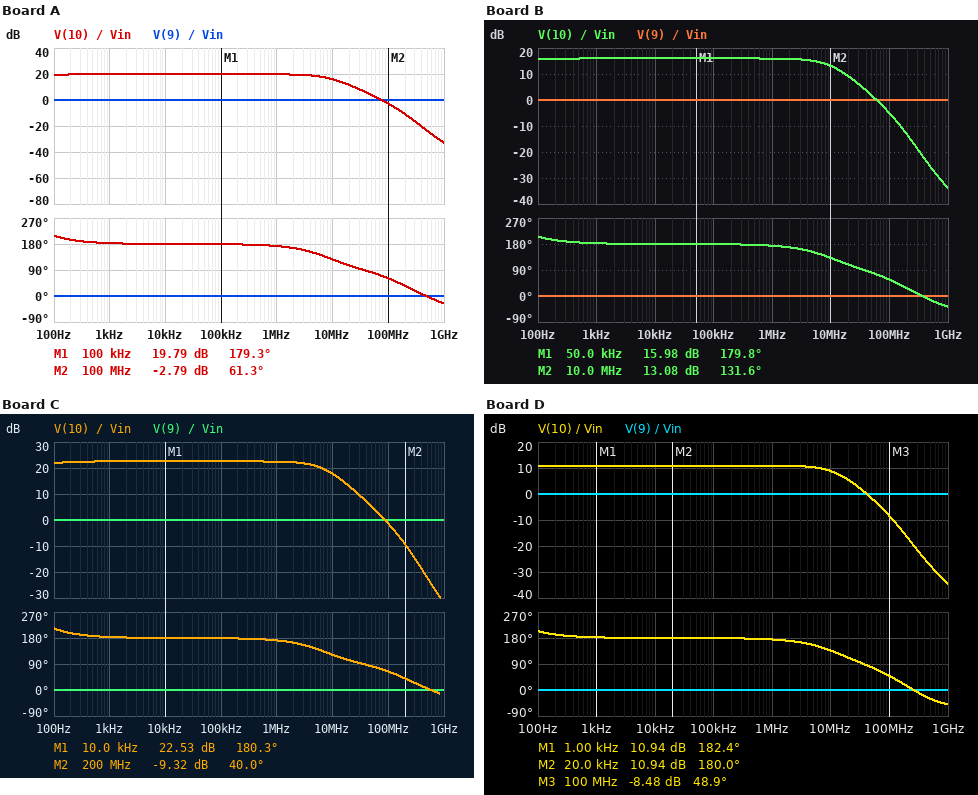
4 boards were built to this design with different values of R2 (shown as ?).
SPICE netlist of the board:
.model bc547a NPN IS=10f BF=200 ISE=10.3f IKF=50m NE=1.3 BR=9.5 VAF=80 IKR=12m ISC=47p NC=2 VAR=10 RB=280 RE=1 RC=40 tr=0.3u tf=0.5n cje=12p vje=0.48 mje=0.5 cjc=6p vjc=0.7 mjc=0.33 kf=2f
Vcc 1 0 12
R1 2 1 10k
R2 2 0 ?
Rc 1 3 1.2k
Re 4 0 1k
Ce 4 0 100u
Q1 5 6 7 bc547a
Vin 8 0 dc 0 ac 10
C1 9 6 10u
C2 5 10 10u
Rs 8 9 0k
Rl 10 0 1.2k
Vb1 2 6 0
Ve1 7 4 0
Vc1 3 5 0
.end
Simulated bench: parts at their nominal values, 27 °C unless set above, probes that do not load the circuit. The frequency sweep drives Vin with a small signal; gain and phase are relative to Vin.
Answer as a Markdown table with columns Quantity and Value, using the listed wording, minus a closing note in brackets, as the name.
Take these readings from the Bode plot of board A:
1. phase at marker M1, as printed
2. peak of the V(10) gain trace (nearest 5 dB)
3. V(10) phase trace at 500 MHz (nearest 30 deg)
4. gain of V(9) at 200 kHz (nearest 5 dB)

| Quantity | Value |
|---|---|
| phase at marker M1, as printed | 179.3 deg |
| peak of the V(10) gain trace | 20 dB |
| V(10) phase trace at 500 MHz | 0 deg |
| gain of V(9) at 200 kHz | 0 dB |
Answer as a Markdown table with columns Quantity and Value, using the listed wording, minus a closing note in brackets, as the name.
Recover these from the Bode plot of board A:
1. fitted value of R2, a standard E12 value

| Quantity | Value |
|---|---|
| fitted value of R2, a standard E12 value | 1 kΩ |
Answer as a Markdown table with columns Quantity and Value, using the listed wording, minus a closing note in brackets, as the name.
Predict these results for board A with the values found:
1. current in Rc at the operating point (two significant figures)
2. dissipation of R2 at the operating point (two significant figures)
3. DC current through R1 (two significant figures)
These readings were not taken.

| Quantity | Value |
|---|---|
| current in Rc at the operating point | 450 µA |
| dissipation of R2 at the operating point | 1.2 mW |
| DC current through R1 | 1.1 mA |
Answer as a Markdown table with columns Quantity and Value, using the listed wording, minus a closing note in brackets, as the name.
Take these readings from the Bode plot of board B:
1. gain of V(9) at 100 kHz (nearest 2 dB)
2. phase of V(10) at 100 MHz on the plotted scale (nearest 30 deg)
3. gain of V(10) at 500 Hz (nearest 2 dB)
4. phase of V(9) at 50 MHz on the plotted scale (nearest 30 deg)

| Quantity | Value |
|---|---|
| gain of V(9) at 100 kHz | 0 dB |
| phase of V(10) at 100 MHz on the plotted scale | 60 deg |
| gain of V(10) at 500 Hz | 16 dB |
| phase of V(9) at 50 MHz on the plotted scale | 0 deg |
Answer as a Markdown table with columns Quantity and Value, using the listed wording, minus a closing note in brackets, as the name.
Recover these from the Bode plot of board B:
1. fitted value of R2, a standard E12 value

| Quantity | Value |
|---|---|
| fitted value of R2, a standard E12 value | 820 Ω |
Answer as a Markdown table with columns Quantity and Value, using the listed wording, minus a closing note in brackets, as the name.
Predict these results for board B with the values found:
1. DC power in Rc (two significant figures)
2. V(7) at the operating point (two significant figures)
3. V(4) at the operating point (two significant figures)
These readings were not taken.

| Quantity | Value |
|---|---|
| DC power in Rc | 96 µW |
| V(7) at the operating point | 290 mV |
| V(4) at the operating point | 290 mV |
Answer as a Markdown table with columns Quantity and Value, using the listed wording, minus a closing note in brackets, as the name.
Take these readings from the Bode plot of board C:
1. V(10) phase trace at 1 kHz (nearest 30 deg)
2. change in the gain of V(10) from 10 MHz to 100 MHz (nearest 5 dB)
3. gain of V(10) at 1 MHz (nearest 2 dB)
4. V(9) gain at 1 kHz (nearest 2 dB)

| Quantity | Value |
|---|---|
| V(10) phase trace at 1 kHz | 180 deg |
| change in the gain of V(10) from 10 MHz to 100 MHz | -20 dB |
| gain of V(10) at 1 MHz | 22 dB |
| V(9) gain at 1 kHz | 0 dB |
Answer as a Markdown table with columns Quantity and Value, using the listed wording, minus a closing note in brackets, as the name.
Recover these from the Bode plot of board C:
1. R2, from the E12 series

| Quantity | Value |
|---|---|
| R2, from the E12 series | 1.2 kΩ |
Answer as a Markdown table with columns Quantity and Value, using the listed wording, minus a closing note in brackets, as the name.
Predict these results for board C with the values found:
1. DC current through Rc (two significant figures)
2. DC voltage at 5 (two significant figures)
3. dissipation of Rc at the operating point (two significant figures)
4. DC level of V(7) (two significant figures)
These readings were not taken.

| Quantity | Value |
|---|---|
| DC current through Rc | 630 µA |
| DC voltage at 5 | 11 V |
| dissipation of Rc at the operating point | 480 µW |
| DC level of V(7) | 640 mV |
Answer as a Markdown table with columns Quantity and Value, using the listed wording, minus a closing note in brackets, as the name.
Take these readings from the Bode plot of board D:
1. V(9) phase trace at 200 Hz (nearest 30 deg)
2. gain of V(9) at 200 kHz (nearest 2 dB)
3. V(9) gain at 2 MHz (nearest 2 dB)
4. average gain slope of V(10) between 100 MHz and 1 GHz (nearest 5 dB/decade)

| Quantity | Value |
|---|---|
| V(9) phase trace at 200 Hz | 0 deg |
| gain of V(9) at 200 kHz | 0 dB |
| V(9) gain at 2 MHz | 0 dB |
| average gain slope of V(10) between 100 MHz and 1 GHz | -25 dB/decade |
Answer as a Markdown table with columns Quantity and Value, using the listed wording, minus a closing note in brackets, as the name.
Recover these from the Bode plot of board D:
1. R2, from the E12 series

| Quantity | Value |
|---|---|
| R2, from the E12 series | 680 Ω |
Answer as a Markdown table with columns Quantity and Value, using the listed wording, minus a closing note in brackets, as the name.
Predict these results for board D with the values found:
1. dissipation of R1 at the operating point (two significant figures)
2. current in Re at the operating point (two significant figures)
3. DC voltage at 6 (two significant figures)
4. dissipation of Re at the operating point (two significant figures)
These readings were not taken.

| Quantity | Value |
|---|---|
| dissipation of R1 at the operating point | 13 mW |
| current in Re at the operating point | 160 µA |
| DC voltage at 6 | 760 mV |
| dissipation of Re at the operating point | 25 µW |
